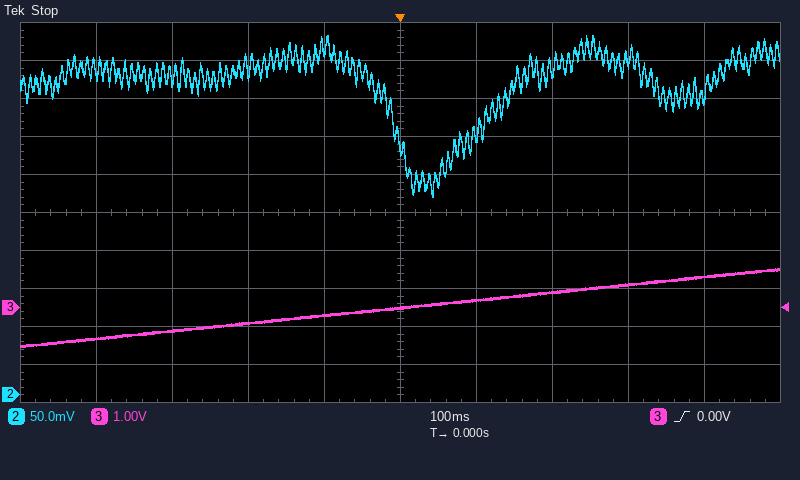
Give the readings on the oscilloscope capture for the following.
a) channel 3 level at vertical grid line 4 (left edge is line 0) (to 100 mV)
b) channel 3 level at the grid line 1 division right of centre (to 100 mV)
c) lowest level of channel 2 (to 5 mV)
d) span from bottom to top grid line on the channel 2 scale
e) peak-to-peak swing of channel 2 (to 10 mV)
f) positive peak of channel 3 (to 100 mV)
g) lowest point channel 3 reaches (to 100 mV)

-200 mV
200 mV
260 mV
500 mV
210 mV
1.0 V
-1.0 V
